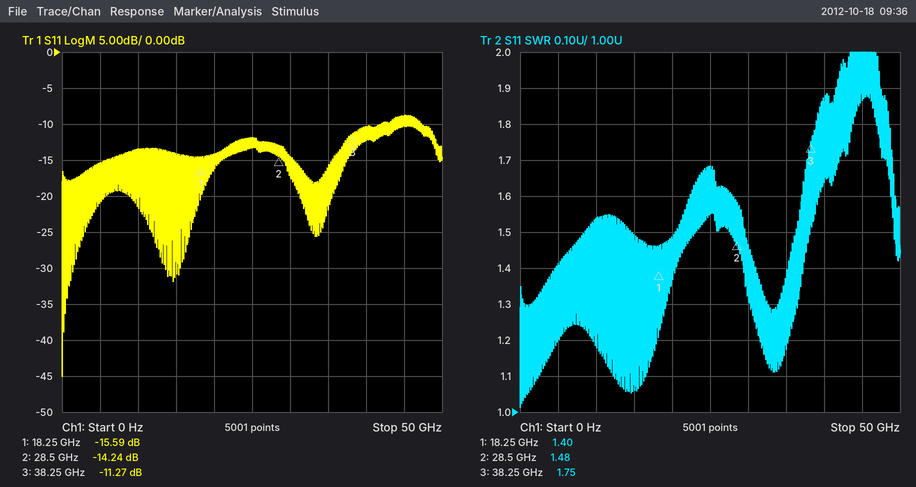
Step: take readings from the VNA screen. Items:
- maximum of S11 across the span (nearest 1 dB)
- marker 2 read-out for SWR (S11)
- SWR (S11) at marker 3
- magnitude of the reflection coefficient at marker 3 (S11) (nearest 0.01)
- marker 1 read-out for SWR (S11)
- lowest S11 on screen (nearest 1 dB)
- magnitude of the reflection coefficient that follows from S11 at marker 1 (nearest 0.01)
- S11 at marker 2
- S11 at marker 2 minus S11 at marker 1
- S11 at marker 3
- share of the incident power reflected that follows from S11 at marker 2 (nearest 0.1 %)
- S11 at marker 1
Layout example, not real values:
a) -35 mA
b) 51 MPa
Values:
a) -9 dB
b) 1.48
c) 1.75
d) 0.27
e) 1.40
f) -45 dB
g) 0.17
h) -14.24 dB
i) 1.35 dB
j) -11.27 dB
k) 3.8 %
l) -15.59 dB
